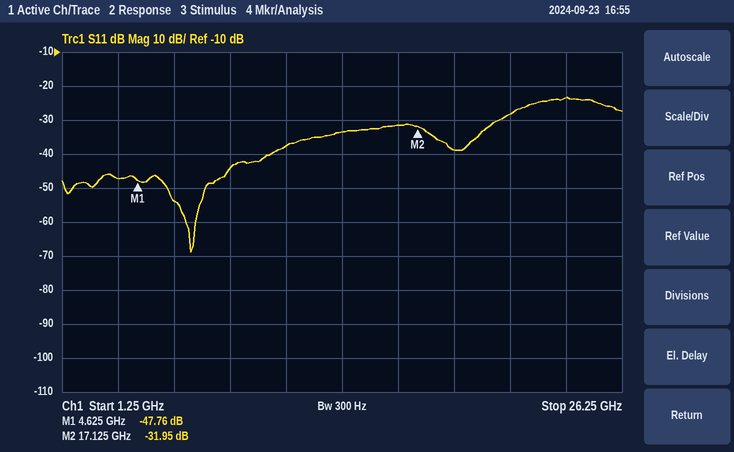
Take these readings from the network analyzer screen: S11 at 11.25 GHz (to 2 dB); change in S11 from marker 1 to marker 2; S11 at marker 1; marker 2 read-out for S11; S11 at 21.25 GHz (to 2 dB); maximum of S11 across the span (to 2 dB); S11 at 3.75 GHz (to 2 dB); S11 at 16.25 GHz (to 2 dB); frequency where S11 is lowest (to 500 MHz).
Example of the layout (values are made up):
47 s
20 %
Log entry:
-38 dB
15.81 dB
-47.76 dB
-31.95 dB
-28 dB
-24 dB
-48 dB
-32 dB
7.0 GHz
